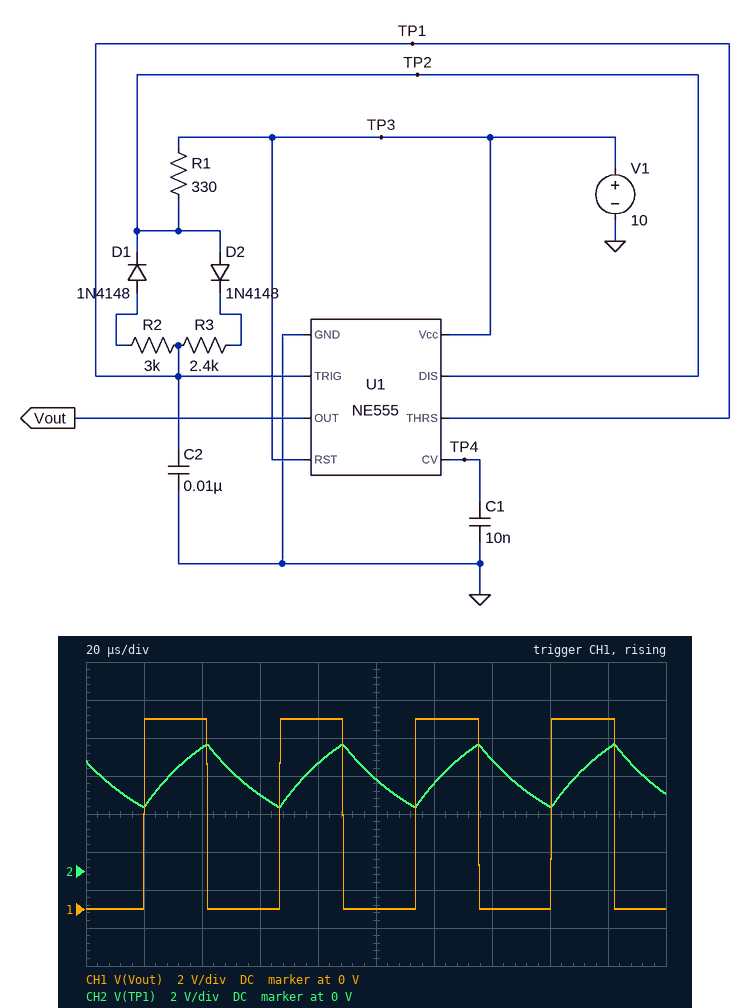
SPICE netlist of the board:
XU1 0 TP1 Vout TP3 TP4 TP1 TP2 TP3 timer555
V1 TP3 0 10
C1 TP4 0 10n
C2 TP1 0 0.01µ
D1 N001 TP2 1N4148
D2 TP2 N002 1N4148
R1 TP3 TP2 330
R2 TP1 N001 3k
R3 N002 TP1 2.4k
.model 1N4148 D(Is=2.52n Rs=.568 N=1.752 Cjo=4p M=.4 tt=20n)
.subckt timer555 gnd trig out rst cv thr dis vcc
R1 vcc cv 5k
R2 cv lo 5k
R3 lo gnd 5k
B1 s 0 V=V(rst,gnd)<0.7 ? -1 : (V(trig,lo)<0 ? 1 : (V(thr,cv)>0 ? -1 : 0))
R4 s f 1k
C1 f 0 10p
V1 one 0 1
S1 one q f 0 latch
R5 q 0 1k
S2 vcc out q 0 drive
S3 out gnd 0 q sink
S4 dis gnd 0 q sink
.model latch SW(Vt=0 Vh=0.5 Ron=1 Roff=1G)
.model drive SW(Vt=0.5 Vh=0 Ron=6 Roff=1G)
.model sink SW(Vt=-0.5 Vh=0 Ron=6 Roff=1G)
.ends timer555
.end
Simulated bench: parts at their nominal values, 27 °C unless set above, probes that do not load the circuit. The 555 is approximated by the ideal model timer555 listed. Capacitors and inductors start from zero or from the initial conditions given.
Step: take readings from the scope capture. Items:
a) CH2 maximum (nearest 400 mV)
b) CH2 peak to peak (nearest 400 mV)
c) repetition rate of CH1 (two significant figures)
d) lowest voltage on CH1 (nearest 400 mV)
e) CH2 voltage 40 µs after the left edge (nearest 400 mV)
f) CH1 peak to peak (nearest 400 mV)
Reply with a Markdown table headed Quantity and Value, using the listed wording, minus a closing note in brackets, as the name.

| Quantity | Value |
|---|---|
| CH2 maximum | 6.8 V |
| CH2 peak to peak | 3.2 V |
| repetition rate of CH1 | 21 kHz |
| lowest voltage on CH1 | 0 V |
| CH2 voltage 40 µs after the left edge | 6.4 V |
| CH1 peak to peak | 10.0 V |
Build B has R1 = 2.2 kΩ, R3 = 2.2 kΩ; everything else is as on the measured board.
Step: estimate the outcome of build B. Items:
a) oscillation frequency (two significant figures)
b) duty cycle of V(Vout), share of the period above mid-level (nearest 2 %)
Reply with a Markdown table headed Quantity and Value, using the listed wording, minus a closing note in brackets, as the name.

| Quantity | Value |
|---|---|
| oscillation frequency | 17 kHz |
| duty cycle of V(Vout), share of the period above mid-level | 60 % |
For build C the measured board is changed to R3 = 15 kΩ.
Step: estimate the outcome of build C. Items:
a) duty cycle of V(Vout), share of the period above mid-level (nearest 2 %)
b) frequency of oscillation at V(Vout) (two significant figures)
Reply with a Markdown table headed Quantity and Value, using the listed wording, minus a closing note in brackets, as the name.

| Quantity | Value |
|---|---|
| duty cycle of V(Vout), share of the period above mid-level | 82 % |
| frequency of oscillation at V(Vout) | 6.9 kHz |
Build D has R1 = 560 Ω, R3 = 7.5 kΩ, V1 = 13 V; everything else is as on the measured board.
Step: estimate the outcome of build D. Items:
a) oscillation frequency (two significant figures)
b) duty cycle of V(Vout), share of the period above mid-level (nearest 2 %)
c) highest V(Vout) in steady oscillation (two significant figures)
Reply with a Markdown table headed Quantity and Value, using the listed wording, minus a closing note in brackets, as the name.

| Quantity | Value |
|---|---|
| oscillation frequency | 12 kHz |
| duty cycle of V(Vout), share of the period above mid-level | 72 % |
| highest V(Vout) in steady oscillation | 13 V |
